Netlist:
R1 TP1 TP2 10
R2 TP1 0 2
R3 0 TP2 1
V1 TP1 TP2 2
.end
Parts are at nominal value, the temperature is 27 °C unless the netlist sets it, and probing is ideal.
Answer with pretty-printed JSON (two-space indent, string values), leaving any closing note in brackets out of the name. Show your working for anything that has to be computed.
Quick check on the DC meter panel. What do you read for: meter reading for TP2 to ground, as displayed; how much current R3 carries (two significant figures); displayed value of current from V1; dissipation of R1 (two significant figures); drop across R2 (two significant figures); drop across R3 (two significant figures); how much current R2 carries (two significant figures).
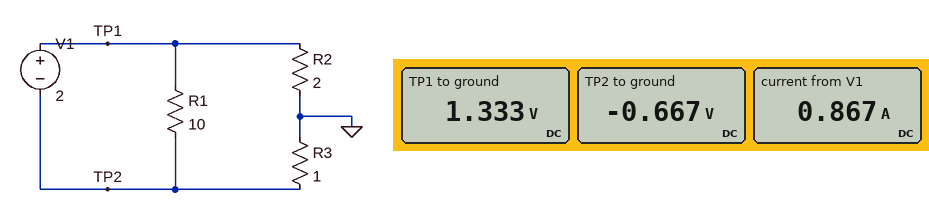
{
  "meter reading for TP2 to ground, as displayed": "-0.667 V",
  "how much current R3 carries": "(0 V - (-667 mV)) / 1 Ω = 670 mA",
  "displayed value of current from V1": "0.867 A",
  "dissipation of R1": "(1.333 V - (-667 mV))^2 / 10 Ω = 400 mW",
  "drop across R2": "1.333 V = 1.3 V",
  "drop across R3": "0 V - (-667 mV) = 670 mV",
  "how much current R2 carries": "(1.333 V) / 2 Ω = 670 mA"
}
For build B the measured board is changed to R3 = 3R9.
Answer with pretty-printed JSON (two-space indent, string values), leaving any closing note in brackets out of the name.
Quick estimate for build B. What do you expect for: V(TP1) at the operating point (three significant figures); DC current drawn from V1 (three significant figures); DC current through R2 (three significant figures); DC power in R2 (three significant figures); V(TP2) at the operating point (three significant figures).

{
  "V(TP1) at the operating point": "678 mV",
  "DC current drawn from V1": "539 mA",
  "DC current through R2": "339 mA",
  "DC power in R2": "230 mW",
  "V(TP2) at the operating point": "-1.32 V"
}
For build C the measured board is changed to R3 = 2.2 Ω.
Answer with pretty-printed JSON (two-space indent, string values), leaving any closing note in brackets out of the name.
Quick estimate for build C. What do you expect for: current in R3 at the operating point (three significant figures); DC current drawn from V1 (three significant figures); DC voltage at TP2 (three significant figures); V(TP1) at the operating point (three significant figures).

{
  "current in R3 at the operating point": "476 mA",
  "DC current drawn from V1": "676 mA",
  "DC voltage at TP2": "-1.05 V",
  "V(TP1) at the operating point": "952 mV"
}
